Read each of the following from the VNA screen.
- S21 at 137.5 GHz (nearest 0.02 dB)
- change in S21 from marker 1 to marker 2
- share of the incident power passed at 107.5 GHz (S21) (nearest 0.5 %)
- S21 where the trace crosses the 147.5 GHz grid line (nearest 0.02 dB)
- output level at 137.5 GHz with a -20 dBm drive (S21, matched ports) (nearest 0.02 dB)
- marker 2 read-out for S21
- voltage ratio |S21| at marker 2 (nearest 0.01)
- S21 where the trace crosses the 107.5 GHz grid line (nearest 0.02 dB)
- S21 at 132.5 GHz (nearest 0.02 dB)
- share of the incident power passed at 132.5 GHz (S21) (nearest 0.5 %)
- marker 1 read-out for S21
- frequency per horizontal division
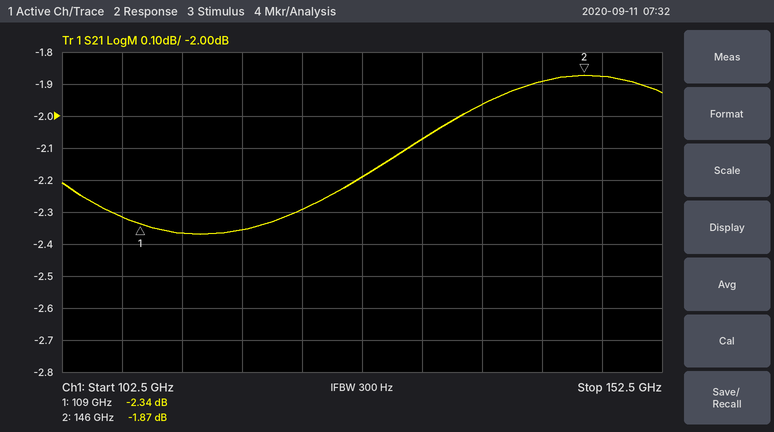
-1.96 dB
0.47 dB
58.5 %
-1.88 dB
-21.96 dBm
-1.87 dB
0.81
-2.32 dB
-2.08 dB
62.0 %
-2.34 dB
5 GHz
